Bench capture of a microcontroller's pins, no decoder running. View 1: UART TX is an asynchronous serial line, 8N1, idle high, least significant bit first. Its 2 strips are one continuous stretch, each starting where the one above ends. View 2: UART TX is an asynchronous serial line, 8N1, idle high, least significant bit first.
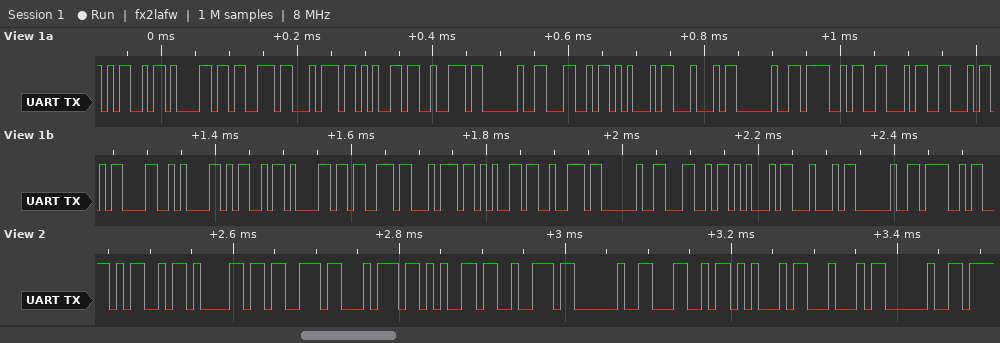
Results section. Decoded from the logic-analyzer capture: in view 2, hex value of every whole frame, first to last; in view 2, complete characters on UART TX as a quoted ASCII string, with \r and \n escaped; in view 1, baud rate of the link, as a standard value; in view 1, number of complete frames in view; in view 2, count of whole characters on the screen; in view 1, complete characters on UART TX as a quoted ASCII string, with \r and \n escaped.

4D 61 73 74 65 72 20 4C 45 44 20
"Master LED "
115200 baud
28
11
"Master LED OFF\r\nMaster LED O"
